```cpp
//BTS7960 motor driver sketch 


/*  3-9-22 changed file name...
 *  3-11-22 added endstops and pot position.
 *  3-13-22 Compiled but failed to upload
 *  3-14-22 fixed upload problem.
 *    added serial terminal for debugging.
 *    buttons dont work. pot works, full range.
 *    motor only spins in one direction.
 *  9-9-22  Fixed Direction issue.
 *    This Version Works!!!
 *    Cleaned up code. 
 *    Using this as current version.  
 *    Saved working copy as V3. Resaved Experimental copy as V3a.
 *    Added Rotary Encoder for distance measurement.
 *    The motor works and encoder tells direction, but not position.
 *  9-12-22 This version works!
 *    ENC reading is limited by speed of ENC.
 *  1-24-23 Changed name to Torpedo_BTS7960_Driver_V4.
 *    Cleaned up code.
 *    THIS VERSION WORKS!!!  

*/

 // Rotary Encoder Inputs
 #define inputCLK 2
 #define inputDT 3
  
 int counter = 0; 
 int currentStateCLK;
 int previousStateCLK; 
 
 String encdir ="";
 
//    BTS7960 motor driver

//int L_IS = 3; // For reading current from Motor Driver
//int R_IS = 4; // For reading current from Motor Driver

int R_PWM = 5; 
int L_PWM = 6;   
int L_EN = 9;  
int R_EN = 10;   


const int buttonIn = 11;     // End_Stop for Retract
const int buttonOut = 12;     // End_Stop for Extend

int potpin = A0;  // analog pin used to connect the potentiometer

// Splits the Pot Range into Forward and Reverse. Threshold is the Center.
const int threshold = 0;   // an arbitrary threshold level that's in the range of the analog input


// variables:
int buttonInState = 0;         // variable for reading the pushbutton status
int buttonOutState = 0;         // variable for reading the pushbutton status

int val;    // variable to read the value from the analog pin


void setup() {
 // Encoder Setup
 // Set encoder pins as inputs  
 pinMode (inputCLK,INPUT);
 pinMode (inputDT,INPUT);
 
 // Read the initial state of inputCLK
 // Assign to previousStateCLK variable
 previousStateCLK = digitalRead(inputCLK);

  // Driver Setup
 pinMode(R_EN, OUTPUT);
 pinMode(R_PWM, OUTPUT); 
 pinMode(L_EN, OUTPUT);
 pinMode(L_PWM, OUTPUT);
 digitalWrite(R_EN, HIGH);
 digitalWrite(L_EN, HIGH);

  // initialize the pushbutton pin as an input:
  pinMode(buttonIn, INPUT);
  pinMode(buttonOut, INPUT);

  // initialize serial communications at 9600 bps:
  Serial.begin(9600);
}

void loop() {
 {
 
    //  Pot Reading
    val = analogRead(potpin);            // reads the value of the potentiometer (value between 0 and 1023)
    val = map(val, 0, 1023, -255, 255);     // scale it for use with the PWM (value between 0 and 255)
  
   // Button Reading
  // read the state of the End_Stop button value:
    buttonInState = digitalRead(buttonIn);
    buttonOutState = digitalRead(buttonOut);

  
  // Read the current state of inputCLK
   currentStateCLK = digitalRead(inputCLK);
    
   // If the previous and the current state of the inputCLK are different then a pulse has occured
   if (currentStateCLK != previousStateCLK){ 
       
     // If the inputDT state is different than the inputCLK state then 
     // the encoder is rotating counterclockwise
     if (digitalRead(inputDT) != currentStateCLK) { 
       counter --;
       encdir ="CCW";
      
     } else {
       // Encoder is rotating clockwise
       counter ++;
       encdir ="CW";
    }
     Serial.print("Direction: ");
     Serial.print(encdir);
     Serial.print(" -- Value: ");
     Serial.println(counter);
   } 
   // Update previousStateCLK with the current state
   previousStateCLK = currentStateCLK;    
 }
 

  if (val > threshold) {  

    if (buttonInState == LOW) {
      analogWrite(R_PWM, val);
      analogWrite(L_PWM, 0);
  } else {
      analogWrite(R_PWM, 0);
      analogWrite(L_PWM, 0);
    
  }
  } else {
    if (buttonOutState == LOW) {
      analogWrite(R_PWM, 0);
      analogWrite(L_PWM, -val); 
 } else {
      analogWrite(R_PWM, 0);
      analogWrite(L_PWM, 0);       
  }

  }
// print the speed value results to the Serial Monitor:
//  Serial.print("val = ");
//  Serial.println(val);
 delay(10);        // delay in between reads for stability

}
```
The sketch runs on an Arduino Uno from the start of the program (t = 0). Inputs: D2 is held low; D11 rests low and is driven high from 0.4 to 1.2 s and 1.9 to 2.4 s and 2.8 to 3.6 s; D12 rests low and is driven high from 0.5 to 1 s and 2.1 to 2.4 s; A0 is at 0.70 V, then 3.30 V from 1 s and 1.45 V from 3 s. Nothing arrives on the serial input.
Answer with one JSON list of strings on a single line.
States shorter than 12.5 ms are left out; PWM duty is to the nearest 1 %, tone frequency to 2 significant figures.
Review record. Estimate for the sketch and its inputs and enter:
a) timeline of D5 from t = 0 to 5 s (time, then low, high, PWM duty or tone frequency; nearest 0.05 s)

["0 s low; 1.2 s PWM 32 %; 1.9 s low; 2.4 s PWM 32 %; 2.8 s low"]
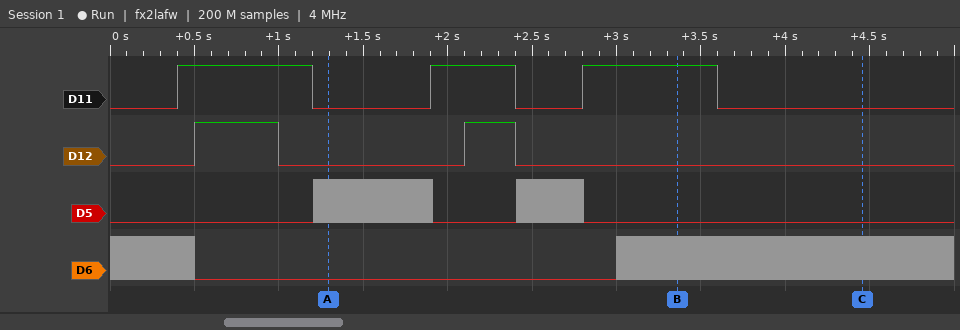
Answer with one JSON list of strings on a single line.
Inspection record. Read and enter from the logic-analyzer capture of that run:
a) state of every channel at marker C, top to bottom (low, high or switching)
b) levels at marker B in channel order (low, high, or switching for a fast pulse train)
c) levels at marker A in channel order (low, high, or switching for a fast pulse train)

["D11 low, D12 low, D5 low, D6 switching", "D11 high, D12 low, D5 low, D6 switching", "D11 low, D12 low, D5 switching, D6 low"]
